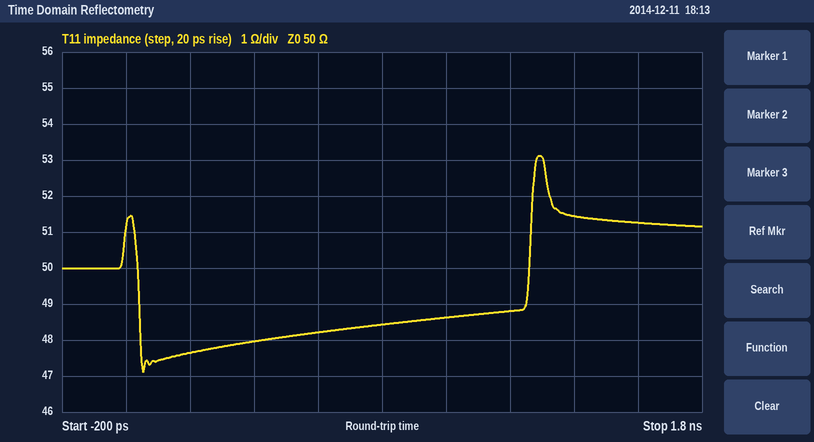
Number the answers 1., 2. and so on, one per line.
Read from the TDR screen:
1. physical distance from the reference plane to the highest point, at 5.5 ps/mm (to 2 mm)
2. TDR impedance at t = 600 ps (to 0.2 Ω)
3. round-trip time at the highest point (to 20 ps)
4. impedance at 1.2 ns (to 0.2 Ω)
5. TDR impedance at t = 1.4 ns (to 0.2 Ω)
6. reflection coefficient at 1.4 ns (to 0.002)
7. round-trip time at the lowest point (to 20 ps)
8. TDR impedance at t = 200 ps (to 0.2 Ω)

1. 118 mm
2. 48.2 Ω
3. 1.30 ns
4. 48.8 Ω
5. 51.4 Ω
6. +0.014
7. 60 ps
8. 47.6 Ω
